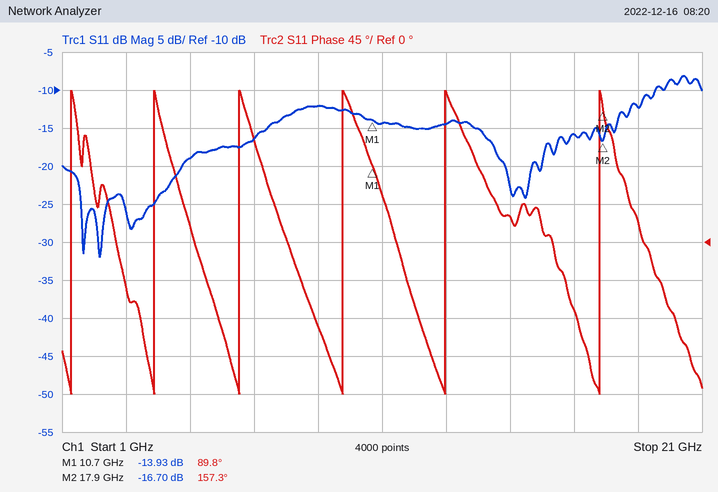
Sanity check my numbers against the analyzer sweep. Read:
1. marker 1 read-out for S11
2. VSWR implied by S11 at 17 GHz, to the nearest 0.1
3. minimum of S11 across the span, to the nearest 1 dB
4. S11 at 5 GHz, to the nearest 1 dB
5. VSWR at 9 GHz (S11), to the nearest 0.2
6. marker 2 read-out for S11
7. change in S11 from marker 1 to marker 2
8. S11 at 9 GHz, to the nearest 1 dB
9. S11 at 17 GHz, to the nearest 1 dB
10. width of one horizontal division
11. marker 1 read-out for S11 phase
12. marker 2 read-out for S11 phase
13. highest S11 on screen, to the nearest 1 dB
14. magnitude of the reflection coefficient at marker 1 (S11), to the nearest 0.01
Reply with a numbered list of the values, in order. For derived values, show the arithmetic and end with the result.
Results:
1. -13.93 dB
2. |Γ| = 10^(-16/20) = 0.1585; VSWR = (1 + 0.1585)/(1 − 0.1585) ≈ 1.4
3. -32 dB
4. -19 dB
5. |Γ| = 10^(-12/20) = 0.2512; VSWR = (1 + 0.2512)/(1 − 0.2512) ≈ 1.67, so 1.6 to the nearest 0.2
6. -16.70 dB
7. -16.7 − (-13.93) = -2.77 dB
8. -12 dB
9. -16 dB
10. 2 GHz
11. 89.8°
12. 157.3°
13. -8 dB
14. 10^(-13.93/20) ≈ 0.20
